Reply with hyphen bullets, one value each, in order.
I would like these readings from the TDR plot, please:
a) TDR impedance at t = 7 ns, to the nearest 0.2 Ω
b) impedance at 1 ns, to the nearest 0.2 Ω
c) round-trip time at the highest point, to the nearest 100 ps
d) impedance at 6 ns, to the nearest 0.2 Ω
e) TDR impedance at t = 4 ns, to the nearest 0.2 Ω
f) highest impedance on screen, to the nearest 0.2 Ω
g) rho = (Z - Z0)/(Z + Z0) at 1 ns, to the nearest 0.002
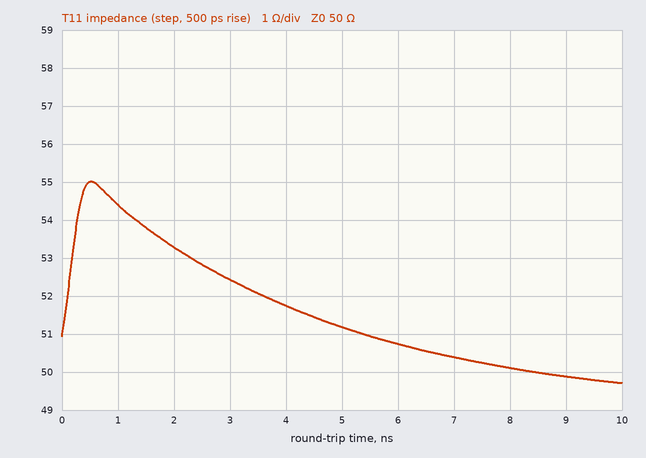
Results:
- 50.4 Ω
- 54.4 Ω
- 500 ps
- 50.8 Ω
- 51.8 Ω
- 55.0 Ω
- +0.042
